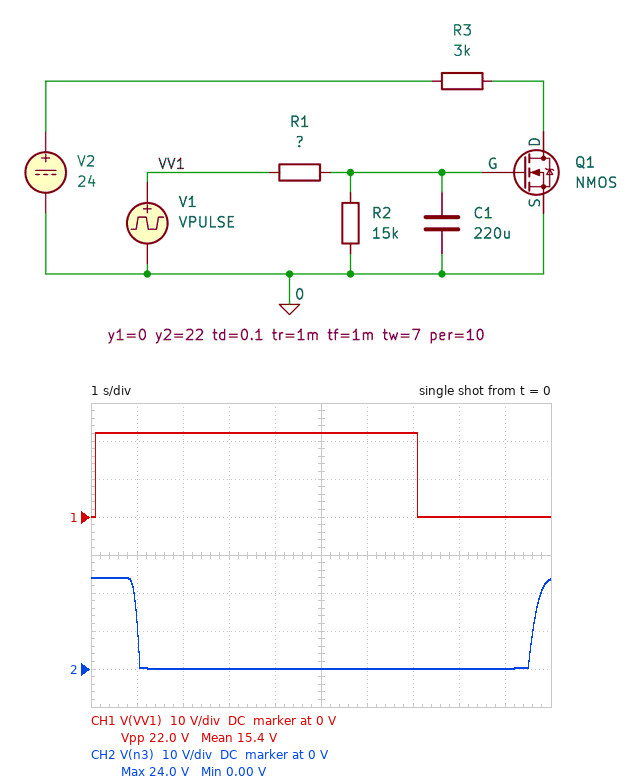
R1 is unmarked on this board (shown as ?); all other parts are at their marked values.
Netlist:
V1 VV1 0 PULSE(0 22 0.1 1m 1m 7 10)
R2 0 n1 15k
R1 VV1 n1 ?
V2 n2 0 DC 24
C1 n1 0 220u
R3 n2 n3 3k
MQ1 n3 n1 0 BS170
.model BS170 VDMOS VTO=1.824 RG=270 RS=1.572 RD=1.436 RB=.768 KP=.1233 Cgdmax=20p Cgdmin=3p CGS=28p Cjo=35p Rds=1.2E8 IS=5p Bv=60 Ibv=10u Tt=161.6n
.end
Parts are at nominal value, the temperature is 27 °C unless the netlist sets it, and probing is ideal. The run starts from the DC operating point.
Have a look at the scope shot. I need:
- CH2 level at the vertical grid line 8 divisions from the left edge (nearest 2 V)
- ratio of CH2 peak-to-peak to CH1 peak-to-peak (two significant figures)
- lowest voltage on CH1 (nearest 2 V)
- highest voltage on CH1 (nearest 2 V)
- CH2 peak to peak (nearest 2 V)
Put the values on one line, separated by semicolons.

0 V; 1.1; 0 V; 22 V; 24 V
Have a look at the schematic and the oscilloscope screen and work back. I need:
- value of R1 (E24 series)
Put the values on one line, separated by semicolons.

36 kΩ
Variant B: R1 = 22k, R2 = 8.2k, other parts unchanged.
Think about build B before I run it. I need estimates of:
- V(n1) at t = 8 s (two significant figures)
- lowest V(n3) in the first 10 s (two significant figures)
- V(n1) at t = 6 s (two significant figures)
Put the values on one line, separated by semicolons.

3.0 V; 40 mV; 5.9 V
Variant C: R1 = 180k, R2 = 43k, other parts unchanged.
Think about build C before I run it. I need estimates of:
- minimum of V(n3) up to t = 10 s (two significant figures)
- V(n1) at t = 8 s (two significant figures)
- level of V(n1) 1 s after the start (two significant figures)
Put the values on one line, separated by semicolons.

120 mV; 2.3 V; 470 mV
